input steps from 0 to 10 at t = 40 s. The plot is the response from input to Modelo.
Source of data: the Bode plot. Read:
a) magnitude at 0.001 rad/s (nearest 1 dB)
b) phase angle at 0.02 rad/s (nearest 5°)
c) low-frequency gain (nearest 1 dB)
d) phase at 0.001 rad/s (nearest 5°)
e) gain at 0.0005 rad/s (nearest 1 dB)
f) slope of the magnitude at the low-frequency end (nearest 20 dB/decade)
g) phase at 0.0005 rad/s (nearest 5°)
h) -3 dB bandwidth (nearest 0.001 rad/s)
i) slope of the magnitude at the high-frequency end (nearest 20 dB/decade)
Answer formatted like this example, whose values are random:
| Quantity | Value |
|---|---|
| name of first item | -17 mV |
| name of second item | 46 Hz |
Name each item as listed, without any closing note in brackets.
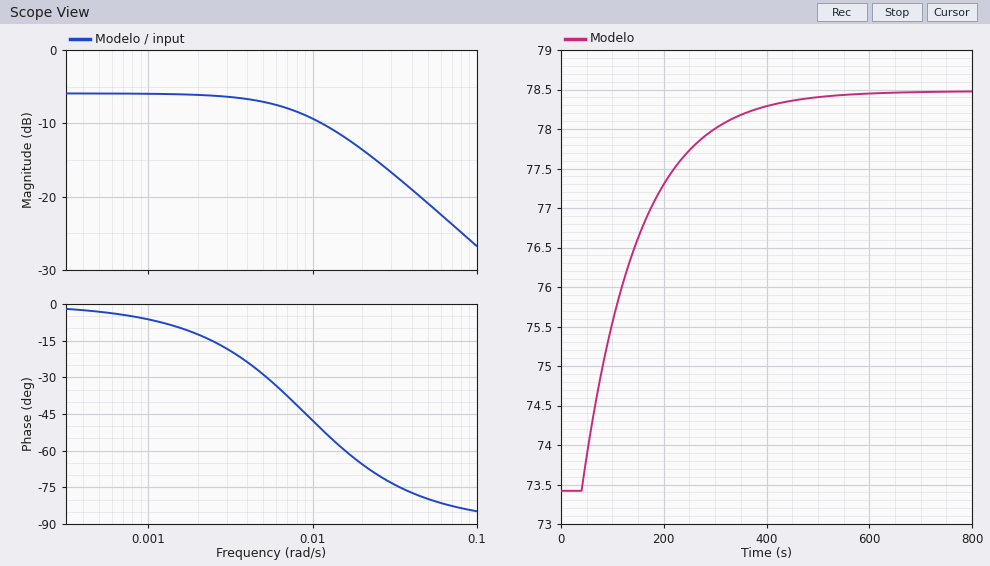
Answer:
| Quantity | Value |
|---|---|
| magnitude at 0.001 rad/s | -6 dB |
| phase angle at 0.02 rad/s | -65° |
| low-frequency gain | -6 dB |
| phase at 0.001 rad/s | -5° |
| gain at 0.0005 rad/s | -6 dB |
| slope of the magnitude at the low-frequency end | 0 dB/decade |
| phase at 0.0005 rad/s | -5° |
| -3 dB bandwidth | 0.009 rad/s |
| slope of the magnitude at the high-frequency end | -20 dB/decade |
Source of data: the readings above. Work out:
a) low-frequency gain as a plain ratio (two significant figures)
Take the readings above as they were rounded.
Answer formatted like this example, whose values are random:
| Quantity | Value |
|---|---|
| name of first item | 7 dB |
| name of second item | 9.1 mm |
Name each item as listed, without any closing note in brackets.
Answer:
| Quantity | Value |
|---|---|
| low-frequency gain as a plain ratio | 0.50 |
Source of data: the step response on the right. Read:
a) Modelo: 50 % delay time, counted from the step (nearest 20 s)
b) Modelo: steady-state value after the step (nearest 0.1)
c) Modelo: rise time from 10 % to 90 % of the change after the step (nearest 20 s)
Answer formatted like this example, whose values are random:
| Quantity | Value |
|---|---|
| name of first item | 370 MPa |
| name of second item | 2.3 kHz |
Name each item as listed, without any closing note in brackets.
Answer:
| Quantity | Value |
|---|---|
| Modelo: 50 % delay time, counted from the step | 80 s |
| Modelo: steady-state value after the step | 78.5 |
| Modelo: rise time from 10 % to 90 % of the change after the step | 240 s |
